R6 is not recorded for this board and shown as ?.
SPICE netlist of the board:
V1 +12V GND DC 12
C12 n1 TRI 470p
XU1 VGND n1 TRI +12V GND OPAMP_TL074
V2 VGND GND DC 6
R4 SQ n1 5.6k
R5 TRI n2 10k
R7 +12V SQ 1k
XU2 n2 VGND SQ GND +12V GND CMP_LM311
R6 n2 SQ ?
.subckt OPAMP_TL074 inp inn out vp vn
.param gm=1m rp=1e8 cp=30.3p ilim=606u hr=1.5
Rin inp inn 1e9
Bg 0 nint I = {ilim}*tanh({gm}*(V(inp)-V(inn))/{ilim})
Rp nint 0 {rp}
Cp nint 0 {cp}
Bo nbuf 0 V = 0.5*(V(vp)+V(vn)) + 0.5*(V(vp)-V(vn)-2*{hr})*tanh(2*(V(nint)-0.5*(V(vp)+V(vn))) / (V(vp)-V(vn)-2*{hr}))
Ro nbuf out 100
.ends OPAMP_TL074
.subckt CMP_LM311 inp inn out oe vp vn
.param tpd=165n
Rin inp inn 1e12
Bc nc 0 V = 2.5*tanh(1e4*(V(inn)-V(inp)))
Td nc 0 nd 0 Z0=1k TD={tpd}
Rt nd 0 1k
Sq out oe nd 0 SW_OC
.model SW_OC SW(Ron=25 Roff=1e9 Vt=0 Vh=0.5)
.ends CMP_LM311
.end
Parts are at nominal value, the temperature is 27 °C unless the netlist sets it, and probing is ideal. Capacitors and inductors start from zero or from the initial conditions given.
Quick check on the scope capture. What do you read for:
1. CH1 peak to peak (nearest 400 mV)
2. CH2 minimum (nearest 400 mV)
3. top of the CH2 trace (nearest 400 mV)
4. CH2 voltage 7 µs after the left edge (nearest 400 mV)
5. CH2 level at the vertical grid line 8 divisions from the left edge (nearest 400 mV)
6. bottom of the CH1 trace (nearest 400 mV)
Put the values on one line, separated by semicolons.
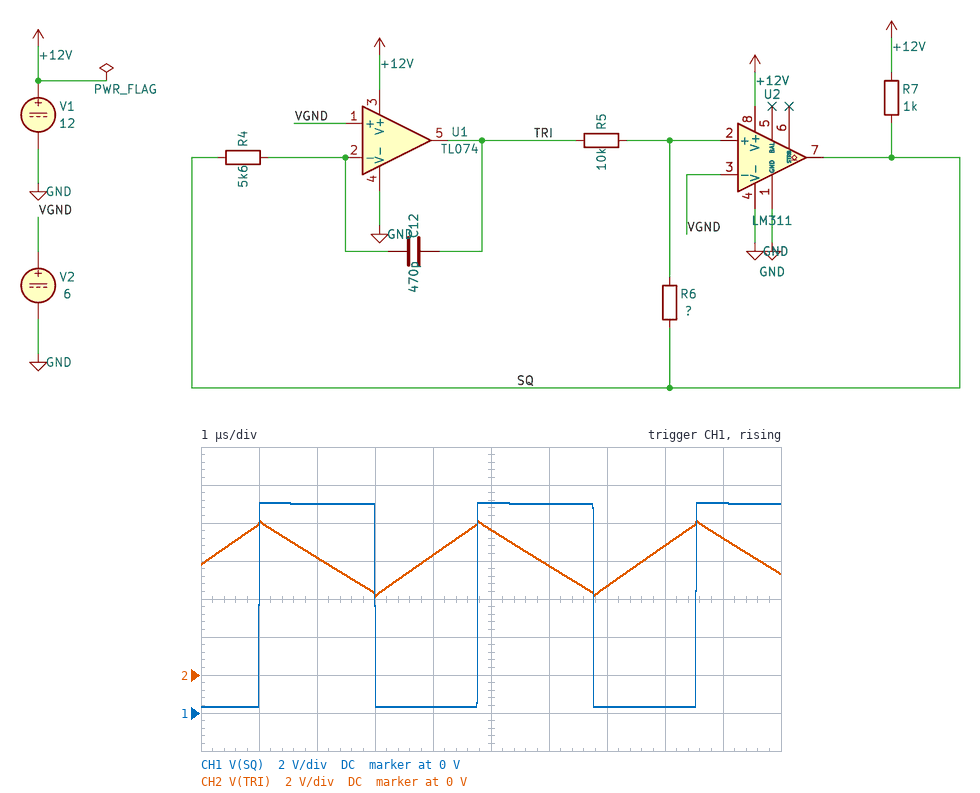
10.8 V; 4.0 V; 8.0 V; 4.8 V; 6.8 V; 400 mV
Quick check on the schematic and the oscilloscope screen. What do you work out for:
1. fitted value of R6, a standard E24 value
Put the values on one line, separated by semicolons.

36 kΩ
